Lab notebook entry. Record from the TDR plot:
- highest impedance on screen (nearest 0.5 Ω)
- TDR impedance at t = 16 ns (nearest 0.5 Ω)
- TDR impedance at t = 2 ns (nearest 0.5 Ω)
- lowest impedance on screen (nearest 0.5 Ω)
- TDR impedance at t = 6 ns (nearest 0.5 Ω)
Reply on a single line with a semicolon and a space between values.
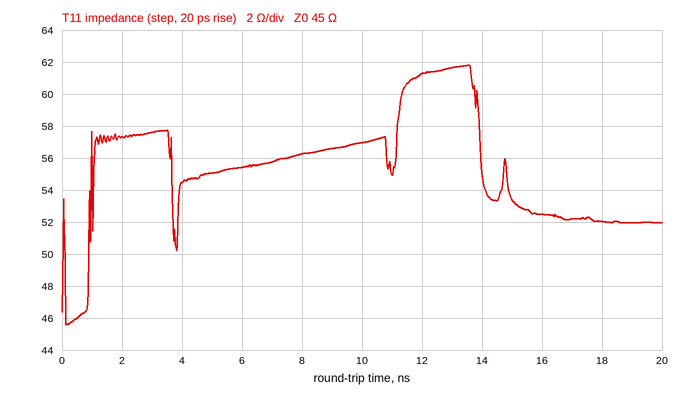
62.0 Ω; 52.5 Ω; 57.5 Ω; 45.5 Ω; 55.5 Ω
